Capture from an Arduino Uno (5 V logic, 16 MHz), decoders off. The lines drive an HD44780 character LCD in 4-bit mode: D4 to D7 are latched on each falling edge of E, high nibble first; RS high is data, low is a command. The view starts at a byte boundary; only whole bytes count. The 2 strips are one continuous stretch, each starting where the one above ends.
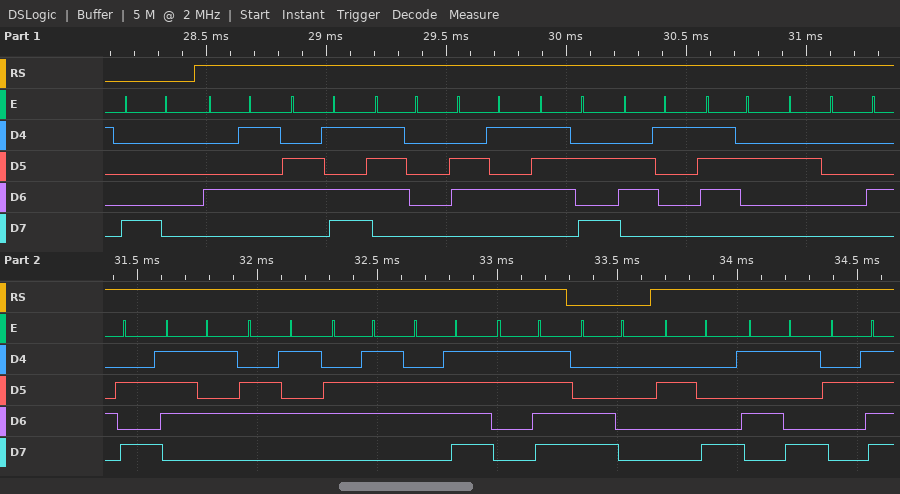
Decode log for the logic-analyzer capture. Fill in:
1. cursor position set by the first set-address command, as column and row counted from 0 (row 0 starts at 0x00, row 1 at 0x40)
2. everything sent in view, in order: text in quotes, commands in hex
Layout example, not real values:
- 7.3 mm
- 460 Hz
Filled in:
- column 0, row 0
- 0x80 "Empezar Juego?" 0xC0 "(Y/"
